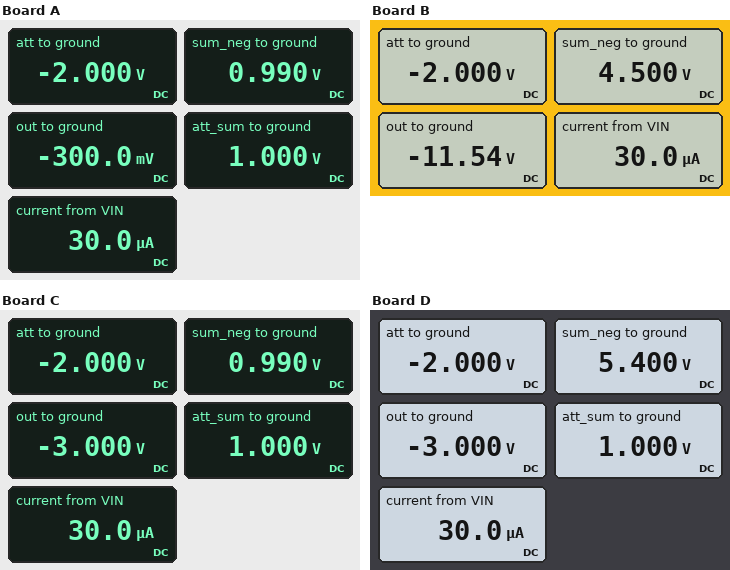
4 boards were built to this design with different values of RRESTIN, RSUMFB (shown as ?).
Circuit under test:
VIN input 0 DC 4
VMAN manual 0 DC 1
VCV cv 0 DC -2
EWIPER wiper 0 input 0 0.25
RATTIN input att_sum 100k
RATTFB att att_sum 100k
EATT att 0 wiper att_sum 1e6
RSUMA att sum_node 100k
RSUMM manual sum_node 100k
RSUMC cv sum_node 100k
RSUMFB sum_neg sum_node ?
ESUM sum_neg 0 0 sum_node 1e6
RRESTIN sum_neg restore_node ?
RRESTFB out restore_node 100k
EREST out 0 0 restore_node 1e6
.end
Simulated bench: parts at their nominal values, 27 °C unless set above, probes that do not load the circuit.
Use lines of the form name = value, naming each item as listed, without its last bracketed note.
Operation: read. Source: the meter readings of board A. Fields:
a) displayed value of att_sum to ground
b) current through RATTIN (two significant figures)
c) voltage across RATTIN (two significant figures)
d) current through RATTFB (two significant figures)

displayed value of att_sum to ground = 1.000 V
current through RATTIN = 30 µA
voltage across RATTIN = 3.0 V
current through RATTFB = 30 µA
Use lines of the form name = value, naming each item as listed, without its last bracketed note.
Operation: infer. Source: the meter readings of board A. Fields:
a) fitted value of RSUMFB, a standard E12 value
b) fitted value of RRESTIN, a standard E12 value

fitted value of RSUMFB, a standard E12 value = 33 kΩ
fitted value of RRESTIN, a standard E12 value = 330 kΩ
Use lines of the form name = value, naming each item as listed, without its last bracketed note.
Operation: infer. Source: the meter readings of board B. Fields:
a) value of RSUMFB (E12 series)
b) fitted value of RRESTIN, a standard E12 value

value of RSUMFB = 150 kΩ
fitted value of RRESTIN, a standard E12 value = 39 kΩ
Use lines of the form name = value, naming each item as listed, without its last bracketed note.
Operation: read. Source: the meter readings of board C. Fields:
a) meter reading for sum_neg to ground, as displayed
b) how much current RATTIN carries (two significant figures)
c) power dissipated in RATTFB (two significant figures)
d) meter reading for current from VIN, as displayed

meter reading for sum_neg to ground, as displayed = 0.990 V
how much current RATTIN carries = 30 µA
power dissipated in RATTFB = 90 µW
meter reading for current from VIN, as displayed = 30.0 µA
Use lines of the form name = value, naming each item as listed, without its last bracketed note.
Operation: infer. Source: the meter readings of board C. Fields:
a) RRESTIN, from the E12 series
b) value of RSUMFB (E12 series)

RRESTIN, from the E12 series = 33 kΩ
value of RSUMFB = 33 kΩ
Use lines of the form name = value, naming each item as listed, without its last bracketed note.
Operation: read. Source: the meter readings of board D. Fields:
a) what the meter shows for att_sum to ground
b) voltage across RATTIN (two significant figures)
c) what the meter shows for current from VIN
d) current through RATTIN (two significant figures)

what the meter shows for att_sum to ground = 1.000 V
voltage across RATTIN = 3.0 V
what the meter shows for current from VIN = 30.0 µA
current through RATTIN = 30 µA
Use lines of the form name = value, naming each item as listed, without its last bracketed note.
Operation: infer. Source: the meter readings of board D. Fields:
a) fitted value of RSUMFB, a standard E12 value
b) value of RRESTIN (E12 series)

fitted value of RSUMFB, a standard E12 value = 180 kΩ
value of RRESTIN = 180 kΩ
